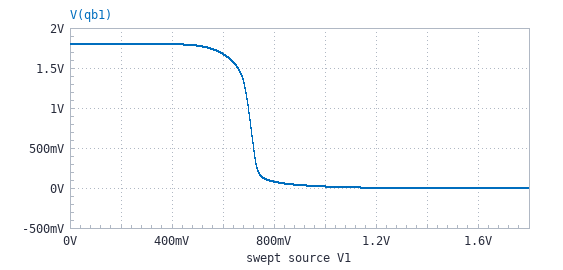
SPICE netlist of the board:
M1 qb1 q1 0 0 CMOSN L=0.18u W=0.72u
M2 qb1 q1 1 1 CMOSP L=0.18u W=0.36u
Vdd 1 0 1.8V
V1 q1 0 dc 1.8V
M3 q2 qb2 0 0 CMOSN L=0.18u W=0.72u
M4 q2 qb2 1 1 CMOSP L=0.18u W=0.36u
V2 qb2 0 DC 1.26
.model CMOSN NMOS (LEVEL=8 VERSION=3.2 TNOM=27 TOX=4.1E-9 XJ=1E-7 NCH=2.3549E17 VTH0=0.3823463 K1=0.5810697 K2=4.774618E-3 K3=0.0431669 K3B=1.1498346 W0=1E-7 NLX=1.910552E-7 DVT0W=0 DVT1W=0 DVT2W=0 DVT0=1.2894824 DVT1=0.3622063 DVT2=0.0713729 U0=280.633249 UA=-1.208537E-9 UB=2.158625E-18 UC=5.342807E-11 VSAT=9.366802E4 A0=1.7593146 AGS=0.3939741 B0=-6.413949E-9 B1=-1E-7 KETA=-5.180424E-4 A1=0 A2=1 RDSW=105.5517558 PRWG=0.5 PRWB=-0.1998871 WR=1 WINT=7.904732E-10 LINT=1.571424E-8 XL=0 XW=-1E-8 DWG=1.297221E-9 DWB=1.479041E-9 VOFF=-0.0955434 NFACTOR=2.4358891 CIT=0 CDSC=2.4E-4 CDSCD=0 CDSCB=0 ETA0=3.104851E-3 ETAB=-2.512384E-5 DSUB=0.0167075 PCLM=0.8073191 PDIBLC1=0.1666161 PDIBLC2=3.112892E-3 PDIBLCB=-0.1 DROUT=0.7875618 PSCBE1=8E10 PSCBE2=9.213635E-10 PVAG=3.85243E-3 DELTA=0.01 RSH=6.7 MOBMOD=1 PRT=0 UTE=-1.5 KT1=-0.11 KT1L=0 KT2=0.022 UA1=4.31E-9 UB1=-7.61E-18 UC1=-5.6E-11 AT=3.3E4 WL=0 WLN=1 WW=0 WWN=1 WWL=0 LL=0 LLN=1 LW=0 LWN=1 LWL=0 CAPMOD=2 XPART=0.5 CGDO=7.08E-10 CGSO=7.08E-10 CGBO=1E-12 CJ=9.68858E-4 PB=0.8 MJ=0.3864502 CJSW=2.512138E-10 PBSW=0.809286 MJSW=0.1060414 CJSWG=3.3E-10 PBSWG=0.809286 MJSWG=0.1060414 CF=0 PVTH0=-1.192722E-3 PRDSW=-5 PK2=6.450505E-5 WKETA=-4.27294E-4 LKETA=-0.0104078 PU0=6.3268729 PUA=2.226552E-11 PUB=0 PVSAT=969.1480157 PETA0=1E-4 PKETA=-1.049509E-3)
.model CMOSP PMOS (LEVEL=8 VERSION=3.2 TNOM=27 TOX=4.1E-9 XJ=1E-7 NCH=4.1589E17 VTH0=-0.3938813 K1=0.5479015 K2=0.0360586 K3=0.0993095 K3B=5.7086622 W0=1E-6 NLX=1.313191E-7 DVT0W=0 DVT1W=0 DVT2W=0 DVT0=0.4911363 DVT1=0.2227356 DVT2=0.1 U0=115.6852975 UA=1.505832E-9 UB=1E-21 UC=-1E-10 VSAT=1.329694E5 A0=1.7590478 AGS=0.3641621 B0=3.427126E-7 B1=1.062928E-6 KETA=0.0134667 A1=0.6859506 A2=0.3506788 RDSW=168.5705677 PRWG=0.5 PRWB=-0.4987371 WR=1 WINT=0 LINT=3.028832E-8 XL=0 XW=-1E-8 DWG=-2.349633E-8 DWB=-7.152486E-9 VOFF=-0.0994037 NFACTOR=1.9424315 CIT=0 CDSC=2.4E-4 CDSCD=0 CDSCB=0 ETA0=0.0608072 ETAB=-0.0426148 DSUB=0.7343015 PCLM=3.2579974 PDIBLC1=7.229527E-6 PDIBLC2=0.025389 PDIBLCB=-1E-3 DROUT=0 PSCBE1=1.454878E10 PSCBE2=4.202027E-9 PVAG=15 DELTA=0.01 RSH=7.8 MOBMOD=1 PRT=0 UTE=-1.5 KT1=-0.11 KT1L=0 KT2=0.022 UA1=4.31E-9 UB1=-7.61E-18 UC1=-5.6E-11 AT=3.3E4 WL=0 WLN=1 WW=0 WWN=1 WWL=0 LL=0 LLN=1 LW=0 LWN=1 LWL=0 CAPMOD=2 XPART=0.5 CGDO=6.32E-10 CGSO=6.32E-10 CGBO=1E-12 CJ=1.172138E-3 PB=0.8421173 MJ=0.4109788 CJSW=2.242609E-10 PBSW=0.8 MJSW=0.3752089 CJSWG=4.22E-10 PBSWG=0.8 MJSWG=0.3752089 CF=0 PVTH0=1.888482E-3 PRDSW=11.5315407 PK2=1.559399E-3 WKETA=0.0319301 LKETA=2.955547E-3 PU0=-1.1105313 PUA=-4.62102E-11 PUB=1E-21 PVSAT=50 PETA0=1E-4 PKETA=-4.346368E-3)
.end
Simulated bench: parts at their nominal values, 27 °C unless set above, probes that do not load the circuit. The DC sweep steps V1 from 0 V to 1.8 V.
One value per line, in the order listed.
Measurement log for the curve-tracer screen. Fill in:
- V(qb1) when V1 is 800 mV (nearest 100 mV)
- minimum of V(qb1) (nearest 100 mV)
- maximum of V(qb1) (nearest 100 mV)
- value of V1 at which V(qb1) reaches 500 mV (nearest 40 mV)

100 mV
0 V
1.8 V
720 mV
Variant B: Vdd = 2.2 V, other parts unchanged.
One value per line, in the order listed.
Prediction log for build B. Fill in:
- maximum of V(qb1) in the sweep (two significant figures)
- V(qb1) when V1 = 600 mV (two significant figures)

2.2 V
2.1 V
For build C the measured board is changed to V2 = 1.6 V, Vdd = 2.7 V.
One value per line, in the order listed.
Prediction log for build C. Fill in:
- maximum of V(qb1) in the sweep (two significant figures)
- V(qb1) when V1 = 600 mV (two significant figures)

2.7 V
2.6 V
